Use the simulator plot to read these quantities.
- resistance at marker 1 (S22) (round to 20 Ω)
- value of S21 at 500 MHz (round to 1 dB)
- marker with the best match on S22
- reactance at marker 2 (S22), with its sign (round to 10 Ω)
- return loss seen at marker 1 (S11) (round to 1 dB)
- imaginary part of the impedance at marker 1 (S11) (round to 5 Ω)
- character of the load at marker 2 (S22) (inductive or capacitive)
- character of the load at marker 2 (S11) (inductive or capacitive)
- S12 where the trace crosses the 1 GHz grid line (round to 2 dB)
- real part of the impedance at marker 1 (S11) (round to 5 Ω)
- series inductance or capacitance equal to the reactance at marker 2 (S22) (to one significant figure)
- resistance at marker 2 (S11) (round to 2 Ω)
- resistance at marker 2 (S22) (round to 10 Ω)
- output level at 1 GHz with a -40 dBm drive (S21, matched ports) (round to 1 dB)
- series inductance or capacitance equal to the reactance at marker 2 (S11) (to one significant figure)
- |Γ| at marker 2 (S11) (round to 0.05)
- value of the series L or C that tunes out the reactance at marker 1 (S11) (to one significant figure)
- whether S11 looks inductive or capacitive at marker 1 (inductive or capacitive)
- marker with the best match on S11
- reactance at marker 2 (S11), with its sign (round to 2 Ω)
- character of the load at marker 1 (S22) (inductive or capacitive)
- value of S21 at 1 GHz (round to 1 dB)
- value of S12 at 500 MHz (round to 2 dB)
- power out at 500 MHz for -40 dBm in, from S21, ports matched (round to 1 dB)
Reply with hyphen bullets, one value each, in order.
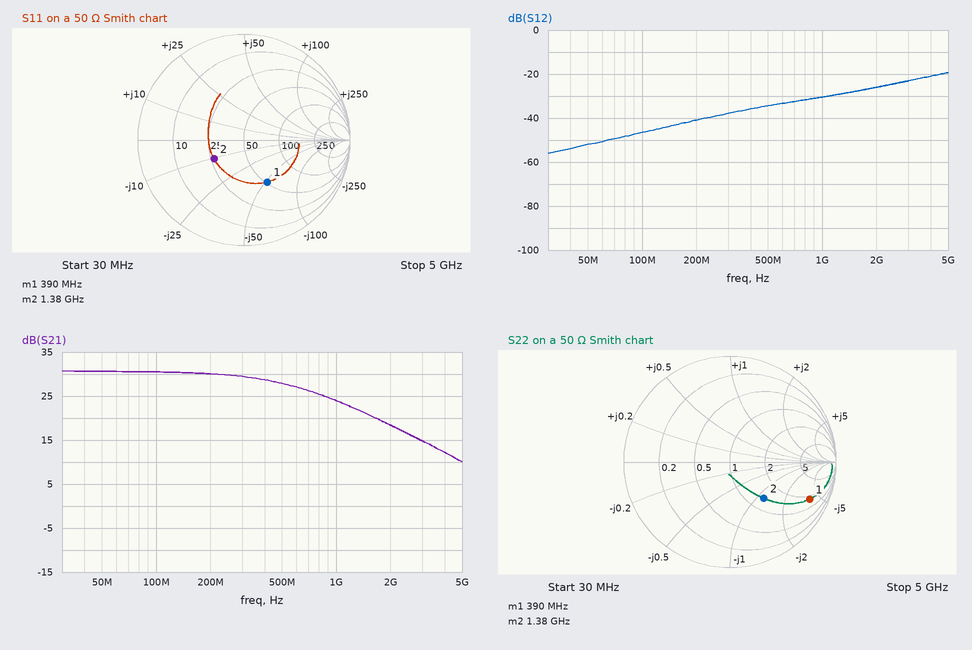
- 80 Ω
- 28 dB
- marker 2
- -60 Ω
- 7 dB
- -50 Ω
- capacitive
- capacitive
- -30 dB
- 50 Ω
- 2 pF
- 26 Ω
- 70 Ω
- -16 dBm
- 10 pF
- 0.35
- 20 nH
- capacitive
- marker 2
- -10 Ω
- capacitive
- 24 dB
- -34 dB
- -12 dBm
